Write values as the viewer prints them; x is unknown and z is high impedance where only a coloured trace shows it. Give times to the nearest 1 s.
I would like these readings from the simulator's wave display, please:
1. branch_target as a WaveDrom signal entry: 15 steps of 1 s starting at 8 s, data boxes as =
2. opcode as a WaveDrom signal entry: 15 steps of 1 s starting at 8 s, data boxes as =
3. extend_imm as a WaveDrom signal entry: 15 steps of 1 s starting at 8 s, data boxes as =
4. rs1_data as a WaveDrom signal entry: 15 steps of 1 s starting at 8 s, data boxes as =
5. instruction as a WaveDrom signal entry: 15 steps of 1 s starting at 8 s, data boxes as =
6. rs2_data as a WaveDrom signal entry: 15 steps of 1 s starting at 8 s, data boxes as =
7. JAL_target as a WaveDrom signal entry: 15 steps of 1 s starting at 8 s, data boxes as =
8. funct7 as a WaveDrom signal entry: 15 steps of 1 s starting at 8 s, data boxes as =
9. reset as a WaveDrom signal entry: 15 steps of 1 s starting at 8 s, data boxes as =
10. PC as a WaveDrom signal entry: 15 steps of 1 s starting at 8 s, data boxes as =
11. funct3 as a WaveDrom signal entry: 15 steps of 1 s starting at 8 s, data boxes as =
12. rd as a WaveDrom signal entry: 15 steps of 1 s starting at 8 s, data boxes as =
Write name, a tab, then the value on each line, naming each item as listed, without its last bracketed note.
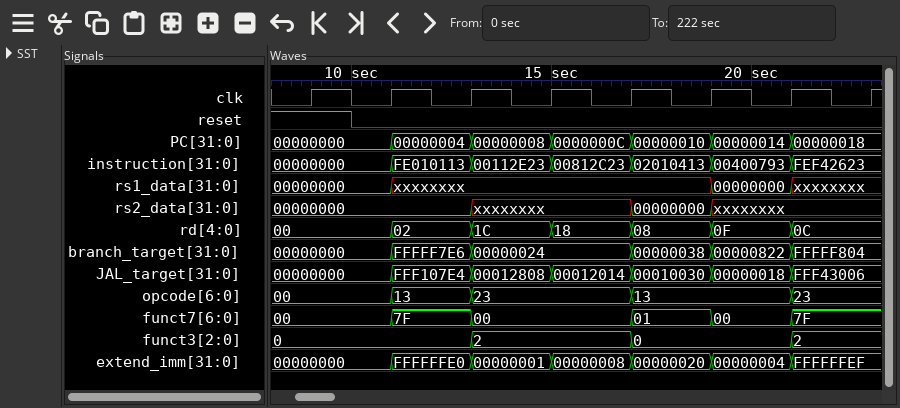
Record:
branch_target as a WaveDrom signal entry: 15 steps of 1 s starting at 8 s, data boxes as =	{name: 'branch_target', wave: '=..=.=...=.=.=.', data: '00000000 FFFFF7E6 00000024 00000038 00000822 FFFFF804'}
opcode as a WaveDrom signal entry: 15 steps of 1 s starting at 8 s, data boxes as =	{name: 'opcode', wave: '=..=.=...=...=.', data: '00 13 23 13 23'}
extend_imm as a WaveDrom signal entry: 15 steps of 1 s starting at 8 s, data boxes as =	{name: 'extend_imm', wave: '=..=.=.=.=.=.=.', data: '00000000 FFFFFFE0 00000001 00000008 00000020 00000004 FFFFFFEF'}
rs1_data as a WaveDrom signal entry: 15 steps of 1 s starting at 8 s, data boxes as =	{name: 'rs1_data', wave: '=..x.......=.x.', data: '00000000 00000000'}
instruction as a WaveDrom signal entry: 15 steps of 1 s starting at 8 s, data boxes as =	{name: 'instruction', wave: '=..=.=.=.=.=.=.', data: '00000000 FE010113 00112E23 00812C23 02010413 00400793 FEF42623'}
rs2_data as a WaveDrom signal entry: 15 steps of 1 s starting at 8 s, data boxes as =	{name: 'rs2_data', wave: '=....x...=.x...', data: '00000000 00000000'}
JAL_target as a WaveDrom signal entry: 15 steps of 1 s starting at 8 s, data boxes as =	{name: 'JAL_target', wave: '=..=.=.=.=.=.=.', data: '00000000 FFF107E4 00012808 00012014 00010030 00000018 FFF43006'}
funct7 as a WaveDrom signal entry: 15 steps of 1 s starting at 8 s, data boxes as =	{name: 'funct7', wave: '=..=.=...=.=.=.', data: '00 7F 00 01 00 7F'}
reset as a WaveDrom signal entry: 15 steps of 1 s starting at 8 s, data boxes as =	{name: 'reset', wave: '1.0............'}
PC as a WaveDrom signal entry: 15 steps of 1 s starting at 8 s, data boxes as =	{name: 'PC', wave: '=..=.=.=.=.=.=.', data: '00000000 00000004 00000008 0000000C 00000010 00000014 00000018'}
funct3 as a WaveDrom signal entry: 15 steps of 1 s starting at 8 s, data boxes as =	{name: 'funct3', wave: '=....=...=...=.', data: '0 2 0 2'}
rd as a WaveDrom signal entry: 15 steps of 1 s starting at 8 s, data boxes as =	{name: 'rd', wave: '=..=.=.=.=.=.=.', data: '00 02 1C 18 08 0F 0C'}
